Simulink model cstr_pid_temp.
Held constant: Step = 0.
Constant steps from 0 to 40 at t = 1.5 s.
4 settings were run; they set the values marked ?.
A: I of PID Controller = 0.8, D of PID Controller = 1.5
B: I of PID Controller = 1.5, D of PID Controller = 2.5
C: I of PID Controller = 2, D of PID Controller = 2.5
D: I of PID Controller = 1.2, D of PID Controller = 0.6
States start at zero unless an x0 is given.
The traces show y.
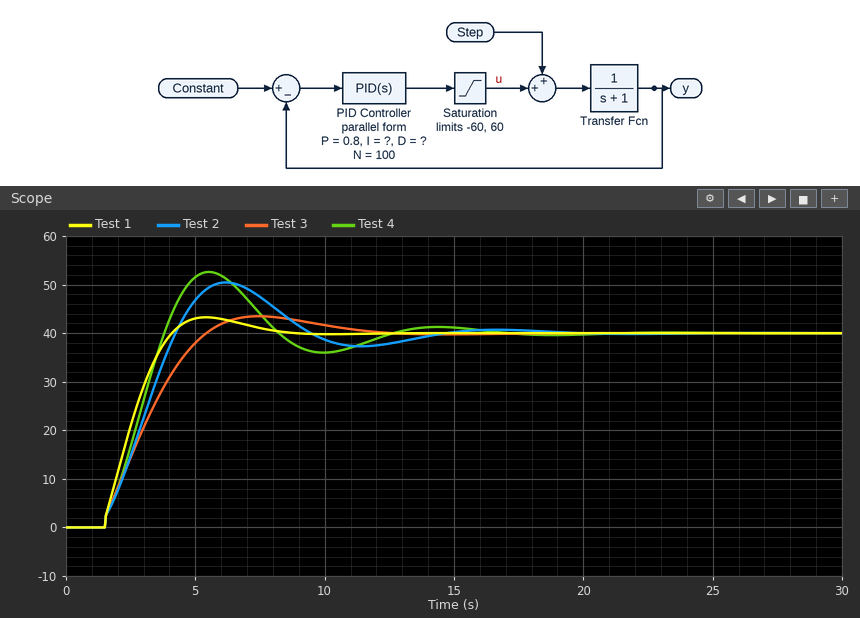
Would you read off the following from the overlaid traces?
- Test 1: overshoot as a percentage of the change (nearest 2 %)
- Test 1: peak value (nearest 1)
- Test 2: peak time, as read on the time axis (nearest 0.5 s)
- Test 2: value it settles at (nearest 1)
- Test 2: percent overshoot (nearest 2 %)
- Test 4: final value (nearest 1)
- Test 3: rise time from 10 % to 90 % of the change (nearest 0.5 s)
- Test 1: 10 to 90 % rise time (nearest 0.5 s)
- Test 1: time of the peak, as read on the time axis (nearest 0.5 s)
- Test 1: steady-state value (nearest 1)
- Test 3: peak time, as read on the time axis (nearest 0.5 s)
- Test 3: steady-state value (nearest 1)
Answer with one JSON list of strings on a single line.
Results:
["8 %", "43", "6.0 s", "40", "26 %", "40", "3.0 s", "2.0 s", "5.5 s", "40", "7.5 s", "40"]
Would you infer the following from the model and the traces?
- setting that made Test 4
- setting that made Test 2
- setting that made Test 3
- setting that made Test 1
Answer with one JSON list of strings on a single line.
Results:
["C", "B", "A", "D"]
